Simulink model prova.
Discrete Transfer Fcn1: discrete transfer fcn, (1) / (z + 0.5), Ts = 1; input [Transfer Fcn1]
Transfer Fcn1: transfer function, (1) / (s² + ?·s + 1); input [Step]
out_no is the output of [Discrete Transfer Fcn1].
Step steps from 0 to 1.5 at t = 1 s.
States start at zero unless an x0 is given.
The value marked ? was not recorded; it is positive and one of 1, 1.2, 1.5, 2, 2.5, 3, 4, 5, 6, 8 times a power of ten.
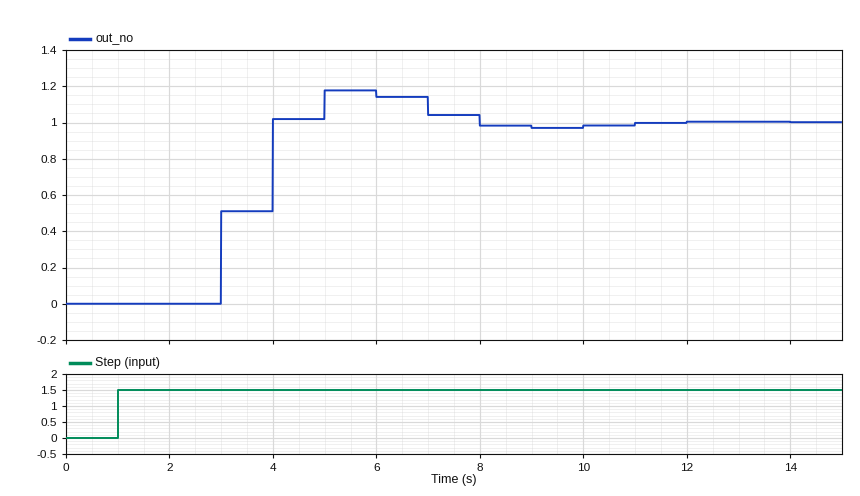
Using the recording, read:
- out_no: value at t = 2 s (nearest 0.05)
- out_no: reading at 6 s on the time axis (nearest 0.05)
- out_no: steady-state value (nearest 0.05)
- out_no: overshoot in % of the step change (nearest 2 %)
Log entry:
0.00
1.15
1.00
18 %
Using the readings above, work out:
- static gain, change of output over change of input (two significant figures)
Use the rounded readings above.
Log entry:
0.67
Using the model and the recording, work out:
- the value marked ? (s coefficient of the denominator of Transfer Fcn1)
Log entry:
1
